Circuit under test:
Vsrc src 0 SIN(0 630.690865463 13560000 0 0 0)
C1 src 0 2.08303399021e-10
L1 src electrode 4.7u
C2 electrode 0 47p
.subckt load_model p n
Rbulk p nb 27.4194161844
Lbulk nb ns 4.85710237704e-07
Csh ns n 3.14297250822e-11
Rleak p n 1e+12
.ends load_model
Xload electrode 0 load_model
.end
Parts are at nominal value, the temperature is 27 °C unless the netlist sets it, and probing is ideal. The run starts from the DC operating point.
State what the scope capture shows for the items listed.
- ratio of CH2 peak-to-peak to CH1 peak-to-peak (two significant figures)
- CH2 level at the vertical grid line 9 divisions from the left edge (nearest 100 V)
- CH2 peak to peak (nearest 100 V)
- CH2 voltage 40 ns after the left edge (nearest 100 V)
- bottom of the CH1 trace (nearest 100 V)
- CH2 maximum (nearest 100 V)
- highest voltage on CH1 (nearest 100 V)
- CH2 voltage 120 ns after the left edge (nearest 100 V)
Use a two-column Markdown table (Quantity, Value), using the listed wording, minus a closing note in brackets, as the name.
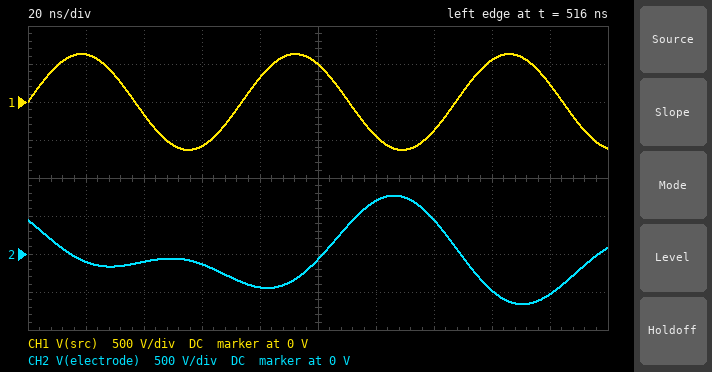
| Quantity | Value |
|---|---|
| ratio of CH2 peak-to-peak to CH1 peak-to-peak | 1.1 |
| CH2 level at the vertical grid line 9 divisions from the left edge | -500 V |
| CH2 peak to peak | 1.4 kV |
| CH2 voltage 40 ns after the left edge | -100 V |
| bottom of the CH1 trace | -600 V |
| CH2 maximum | 800 V |
| highest voltage on CH1 | 600 V |
| CH2 voltage 120 ns after the left edge | 700 V |
